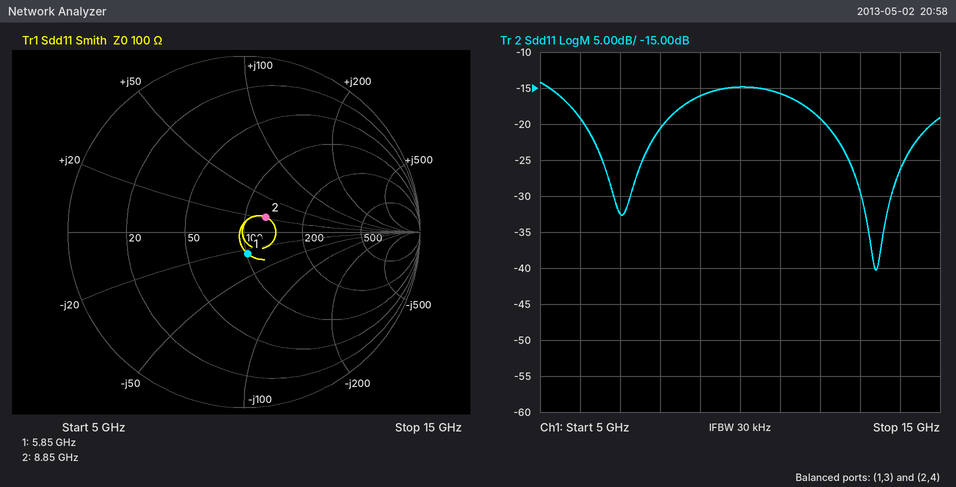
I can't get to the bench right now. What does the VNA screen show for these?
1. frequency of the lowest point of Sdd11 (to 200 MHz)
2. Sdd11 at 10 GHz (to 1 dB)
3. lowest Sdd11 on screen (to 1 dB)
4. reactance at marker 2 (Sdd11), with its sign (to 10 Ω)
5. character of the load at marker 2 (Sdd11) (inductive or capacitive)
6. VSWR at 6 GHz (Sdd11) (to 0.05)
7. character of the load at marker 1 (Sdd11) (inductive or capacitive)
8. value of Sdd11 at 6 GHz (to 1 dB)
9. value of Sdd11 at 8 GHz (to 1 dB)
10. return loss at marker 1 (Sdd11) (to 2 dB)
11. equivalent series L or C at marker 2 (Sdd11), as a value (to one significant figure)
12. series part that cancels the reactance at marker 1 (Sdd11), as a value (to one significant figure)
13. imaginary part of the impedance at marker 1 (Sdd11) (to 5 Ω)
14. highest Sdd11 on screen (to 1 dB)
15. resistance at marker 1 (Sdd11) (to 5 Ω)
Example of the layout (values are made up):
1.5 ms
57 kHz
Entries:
13.4 GHz
-15 dB
-40 dB
+20 Ω
inductive
1.25
capacitive
-19 dB
-21 dB
18 dB
400 pH
700 pH
-25 Ω
-14 dB
100 Ω
